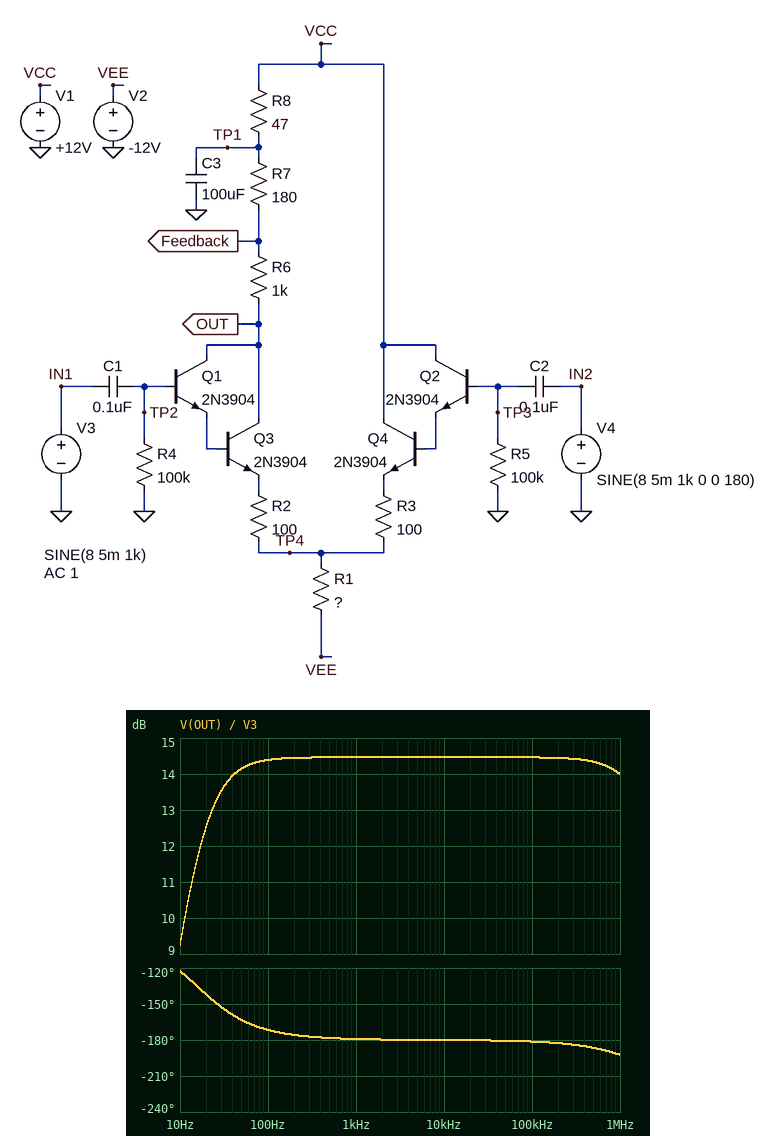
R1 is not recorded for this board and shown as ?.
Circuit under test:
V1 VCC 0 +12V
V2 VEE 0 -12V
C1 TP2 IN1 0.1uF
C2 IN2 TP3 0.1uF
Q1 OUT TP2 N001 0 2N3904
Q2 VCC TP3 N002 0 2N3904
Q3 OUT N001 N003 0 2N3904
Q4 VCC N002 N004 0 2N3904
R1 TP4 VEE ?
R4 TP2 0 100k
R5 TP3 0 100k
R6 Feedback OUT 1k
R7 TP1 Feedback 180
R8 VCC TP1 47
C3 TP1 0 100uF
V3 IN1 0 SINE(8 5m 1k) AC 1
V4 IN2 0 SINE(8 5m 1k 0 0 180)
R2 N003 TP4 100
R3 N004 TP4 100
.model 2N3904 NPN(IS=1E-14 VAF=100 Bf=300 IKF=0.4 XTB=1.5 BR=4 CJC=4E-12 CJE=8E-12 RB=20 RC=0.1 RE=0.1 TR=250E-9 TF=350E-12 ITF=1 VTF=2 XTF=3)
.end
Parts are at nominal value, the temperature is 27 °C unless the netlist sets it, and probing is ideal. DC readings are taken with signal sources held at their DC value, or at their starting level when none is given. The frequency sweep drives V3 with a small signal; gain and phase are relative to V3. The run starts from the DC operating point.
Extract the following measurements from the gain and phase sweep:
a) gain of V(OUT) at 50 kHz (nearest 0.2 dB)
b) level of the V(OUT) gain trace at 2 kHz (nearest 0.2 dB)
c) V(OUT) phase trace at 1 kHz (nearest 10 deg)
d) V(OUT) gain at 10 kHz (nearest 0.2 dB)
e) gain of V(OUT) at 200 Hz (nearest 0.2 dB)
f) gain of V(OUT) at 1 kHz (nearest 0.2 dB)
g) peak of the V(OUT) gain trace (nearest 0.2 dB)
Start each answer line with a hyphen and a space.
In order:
- 14.4 dB
- 14.4 dB
- -180 deg
- 14.4 dB
- 14.4 dB
- 14.4 dB
- 14.4 dB
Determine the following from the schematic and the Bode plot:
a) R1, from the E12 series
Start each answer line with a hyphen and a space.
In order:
- 1.5 kΩ
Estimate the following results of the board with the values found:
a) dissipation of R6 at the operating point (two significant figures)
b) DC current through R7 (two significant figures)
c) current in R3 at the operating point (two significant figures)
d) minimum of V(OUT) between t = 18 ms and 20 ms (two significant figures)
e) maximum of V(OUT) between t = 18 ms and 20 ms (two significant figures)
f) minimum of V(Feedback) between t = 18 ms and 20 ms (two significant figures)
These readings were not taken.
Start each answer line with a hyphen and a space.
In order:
- 12 mW
- 3.5 mA
- 3.5 mA
- 7.7 V
- 7.8 V
- 11 V
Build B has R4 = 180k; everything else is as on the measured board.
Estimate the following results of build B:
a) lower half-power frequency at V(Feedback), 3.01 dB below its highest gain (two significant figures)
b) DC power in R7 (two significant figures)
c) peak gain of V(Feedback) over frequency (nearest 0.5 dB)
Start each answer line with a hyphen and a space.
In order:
- 7.2 Hz
- 2.1 mW
- -1.0 dB
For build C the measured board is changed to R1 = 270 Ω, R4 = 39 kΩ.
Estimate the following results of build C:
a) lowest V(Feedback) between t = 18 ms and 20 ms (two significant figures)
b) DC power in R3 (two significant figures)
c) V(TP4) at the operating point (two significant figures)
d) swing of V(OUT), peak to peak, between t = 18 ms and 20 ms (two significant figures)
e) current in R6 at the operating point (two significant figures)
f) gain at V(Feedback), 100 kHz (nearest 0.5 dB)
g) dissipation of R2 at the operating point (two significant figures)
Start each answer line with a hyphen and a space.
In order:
- 9.5 V
- 43 mW
- -3.4 V
- 6.8 mV
- 11 mA
- -33.5 dB
- 12 mW
